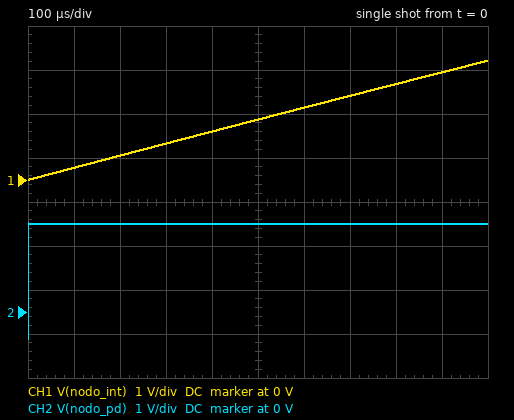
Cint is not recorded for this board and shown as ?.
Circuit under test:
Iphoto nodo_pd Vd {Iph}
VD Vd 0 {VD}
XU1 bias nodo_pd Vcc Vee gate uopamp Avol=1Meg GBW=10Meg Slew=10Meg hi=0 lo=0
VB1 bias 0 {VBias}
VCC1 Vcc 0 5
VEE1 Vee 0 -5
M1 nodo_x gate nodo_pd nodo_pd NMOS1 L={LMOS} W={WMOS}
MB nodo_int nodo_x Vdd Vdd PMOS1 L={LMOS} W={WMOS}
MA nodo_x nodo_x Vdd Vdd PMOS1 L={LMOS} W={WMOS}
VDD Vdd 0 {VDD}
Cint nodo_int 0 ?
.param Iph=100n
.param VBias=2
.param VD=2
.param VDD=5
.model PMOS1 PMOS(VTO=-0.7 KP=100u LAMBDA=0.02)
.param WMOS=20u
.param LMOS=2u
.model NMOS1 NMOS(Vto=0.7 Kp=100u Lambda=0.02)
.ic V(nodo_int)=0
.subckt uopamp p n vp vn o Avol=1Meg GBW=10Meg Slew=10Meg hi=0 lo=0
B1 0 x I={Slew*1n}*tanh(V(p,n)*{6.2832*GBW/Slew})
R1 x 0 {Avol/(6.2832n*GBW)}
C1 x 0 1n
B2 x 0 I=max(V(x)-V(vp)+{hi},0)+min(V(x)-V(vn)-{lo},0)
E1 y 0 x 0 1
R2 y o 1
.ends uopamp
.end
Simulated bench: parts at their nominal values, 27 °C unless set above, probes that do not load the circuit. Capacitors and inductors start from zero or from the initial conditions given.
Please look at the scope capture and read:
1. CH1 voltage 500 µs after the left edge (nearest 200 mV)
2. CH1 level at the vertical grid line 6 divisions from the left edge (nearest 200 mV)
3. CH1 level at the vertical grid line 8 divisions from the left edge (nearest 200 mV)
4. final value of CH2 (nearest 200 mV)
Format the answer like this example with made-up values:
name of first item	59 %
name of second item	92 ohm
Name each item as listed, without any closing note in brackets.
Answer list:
CH1 voltage 500 µs after the left edge	1.4 V
CH1 level at the vertical grid line 6 divisions from the left edge	1.6 V
CH1 level at the vertical grid line 8 divisions from the left edge	2.2 V
final value of CH2	2.0 V
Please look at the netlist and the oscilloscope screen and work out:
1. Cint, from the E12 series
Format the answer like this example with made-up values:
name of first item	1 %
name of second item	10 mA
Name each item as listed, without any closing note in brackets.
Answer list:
Cint, from the E12 series	39 pF
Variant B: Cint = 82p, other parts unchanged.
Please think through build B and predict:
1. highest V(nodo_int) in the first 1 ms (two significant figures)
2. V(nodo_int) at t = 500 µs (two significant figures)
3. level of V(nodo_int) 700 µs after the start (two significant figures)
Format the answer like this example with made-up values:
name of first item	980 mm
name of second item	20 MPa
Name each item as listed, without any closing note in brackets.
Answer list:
highest V(nodo_int) in the first 1 ms	1.3 V
V(nodo_int) at t = 500 µs	660 mV
level of V(nodo_int) 700 µs after the start	920 mV
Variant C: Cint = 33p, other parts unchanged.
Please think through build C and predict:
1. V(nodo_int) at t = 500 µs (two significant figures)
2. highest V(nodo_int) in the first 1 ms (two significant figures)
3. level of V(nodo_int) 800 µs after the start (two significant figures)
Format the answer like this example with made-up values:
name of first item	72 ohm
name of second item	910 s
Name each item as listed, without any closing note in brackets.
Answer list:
V(nodo_int) at t = 500 µs	1.6 V
highest V(nodo_int) in the first 1 ms	3.2 V
level of V(nodo_int) 800 µs after the start	2.6 V
